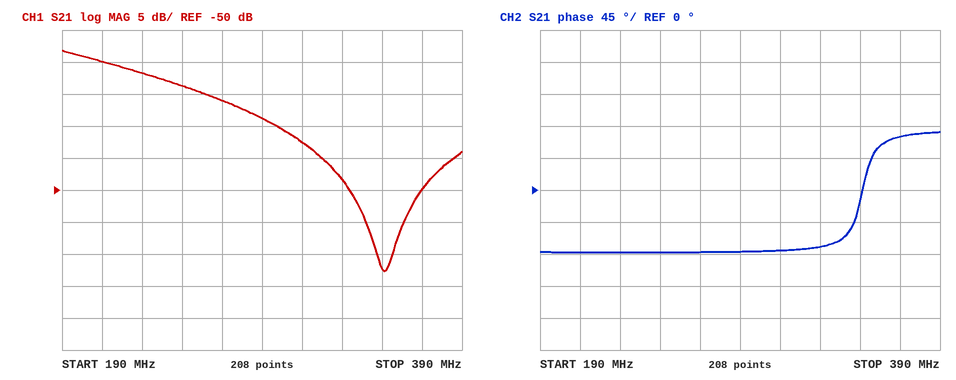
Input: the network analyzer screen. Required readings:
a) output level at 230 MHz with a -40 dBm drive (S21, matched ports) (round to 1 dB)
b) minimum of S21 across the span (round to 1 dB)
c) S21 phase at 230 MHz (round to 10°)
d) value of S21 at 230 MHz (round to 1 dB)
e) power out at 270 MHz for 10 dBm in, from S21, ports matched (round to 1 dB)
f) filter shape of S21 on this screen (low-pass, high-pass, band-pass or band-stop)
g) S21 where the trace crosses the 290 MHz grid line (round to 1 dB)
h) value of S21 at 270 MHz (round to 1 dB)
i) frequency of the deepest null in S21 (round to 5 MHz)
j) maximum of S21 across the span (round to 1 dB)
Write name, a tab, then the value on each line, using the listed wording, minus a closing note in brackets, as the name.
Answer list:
output level at 230 MHz with a -40 dBm drive (S21, matched ports)	-72 dBm
minimum of S21 across the span	-63 dB
S21 phase at 230 MHz	-90°
value of S21 at 230 MHz	-32 dB
power out at 270 MHz for 10 dBm in, from S21, ports matched	-26 dBm
filter shape of S21 on this screen	low-pass
S21 where the trace crosses the 290 MHz grid line	-39 dB
value of S21 at 270 MHz	-36 dB
frequency of the deepest null in S21	350 MHz
maximum of S21 across the span	-28 dB
